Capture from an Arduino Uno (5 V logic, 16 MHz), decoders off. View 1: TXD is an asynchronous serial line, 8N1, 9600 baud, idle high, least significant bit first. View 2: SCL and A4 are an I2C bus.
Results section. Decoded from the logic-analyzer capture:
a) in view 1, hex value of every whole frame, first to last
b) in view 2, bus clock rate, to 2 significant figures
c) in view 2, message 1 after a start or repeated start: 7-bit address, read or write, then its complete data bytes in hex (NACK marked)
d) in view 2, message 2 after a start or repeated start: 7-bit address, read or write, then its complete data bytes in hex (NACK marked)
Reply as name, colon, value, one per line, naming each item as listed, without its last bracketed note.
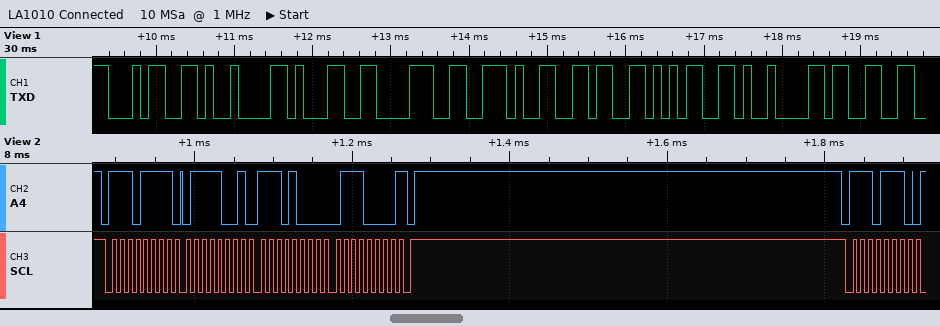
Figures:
in view 1, hex value of every whole frame, first to last: 0x34 0x09 0x31 0x38 0x2E 0x36 0x35 0x09 0x33
in view 2, bus clock rate, to 2 significant figures: 100 kHz
in view 2, message 1 after a start or repeated start: 7-bit address, read or write, then its complete data bytes in hex: 0x77 read: 79 E8 70 NACK
in view 2, message 2 after a start or repeated start: 7-bit address, read or write, then its complete data bytes in hex: 0x77 write
